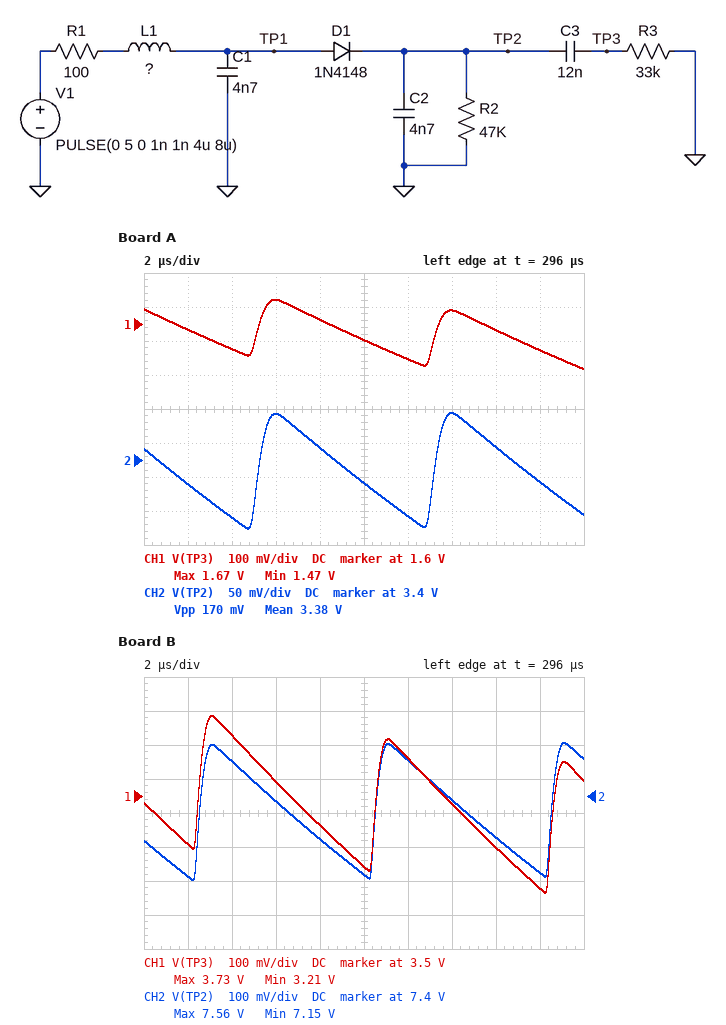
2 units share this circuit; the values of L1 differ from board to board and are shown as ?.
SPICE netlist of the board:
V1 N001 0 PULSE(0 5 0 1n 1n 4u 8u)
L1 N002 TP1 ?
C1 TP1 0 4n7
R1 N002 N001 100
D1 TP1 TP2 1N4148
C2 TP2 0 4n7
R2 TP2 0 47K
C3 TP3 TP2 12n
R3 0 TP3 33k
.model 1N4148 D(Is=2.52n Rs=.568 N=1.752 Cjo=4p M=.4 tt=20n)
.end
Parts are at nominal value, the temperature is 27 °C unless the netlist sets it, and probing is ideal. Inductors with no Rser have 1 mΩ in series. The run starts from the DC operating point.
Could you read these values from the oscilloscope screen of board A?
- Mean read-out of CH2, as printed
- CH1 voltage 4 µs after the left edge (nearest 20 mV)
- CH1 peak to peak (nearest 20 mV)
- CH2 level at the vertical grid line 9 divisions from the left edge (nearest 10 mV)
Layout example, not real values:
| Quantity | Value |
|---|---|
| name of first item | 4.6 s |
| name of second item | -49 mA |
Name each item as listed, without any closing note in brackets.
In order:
| Quantity | Value |
|---|---|
| Mean read-out of CH2, as printed | 3.38 V |
| CH1 voltage 4 µs after the left edge | 1.52 V |
| CH1 peak to peak | 200 mV |
| CH2 level at the vertical grid line 9 divisions from the left edge | 3.37 V |
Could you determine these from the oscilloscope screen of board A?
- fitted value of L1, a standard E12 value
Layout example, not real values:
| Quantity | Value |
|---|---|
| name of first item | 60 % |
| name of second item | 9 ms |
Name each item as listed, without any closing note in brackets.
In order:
| Quantity | Value |
|---|---|
| fitted value of L1, a standard E12 value | 1 mH |
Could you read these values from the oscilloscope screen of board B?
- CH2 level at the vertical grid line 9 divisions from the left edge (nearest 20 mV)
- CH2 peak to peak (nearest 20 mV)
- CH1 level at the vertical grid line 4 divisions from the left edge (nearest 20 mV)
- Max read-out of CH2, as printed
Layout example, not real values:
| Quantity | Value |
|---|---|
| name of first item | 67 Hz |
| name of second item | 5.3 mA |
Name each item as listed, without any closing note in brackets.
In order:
| Quantity | Value |
|---|---|
| CH2 level at the vertical grid line 9 divisions from the left edge | 7.18 V |
| CH2 peak to peak | 400 mV |
| CH1 level at the vertical grid line 4 divisions from the left edge | 3.42 V |
| Max read-out of CH2, as printed | 7.56 V |
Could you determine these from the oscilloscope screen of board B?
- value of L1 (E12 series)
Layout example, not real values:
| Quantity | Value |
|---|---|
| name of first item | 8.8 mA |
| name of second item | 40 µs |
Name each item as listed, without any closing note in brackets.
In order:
| Quantity | Value |
|---|---|
| value of L1 | 220 µH |
